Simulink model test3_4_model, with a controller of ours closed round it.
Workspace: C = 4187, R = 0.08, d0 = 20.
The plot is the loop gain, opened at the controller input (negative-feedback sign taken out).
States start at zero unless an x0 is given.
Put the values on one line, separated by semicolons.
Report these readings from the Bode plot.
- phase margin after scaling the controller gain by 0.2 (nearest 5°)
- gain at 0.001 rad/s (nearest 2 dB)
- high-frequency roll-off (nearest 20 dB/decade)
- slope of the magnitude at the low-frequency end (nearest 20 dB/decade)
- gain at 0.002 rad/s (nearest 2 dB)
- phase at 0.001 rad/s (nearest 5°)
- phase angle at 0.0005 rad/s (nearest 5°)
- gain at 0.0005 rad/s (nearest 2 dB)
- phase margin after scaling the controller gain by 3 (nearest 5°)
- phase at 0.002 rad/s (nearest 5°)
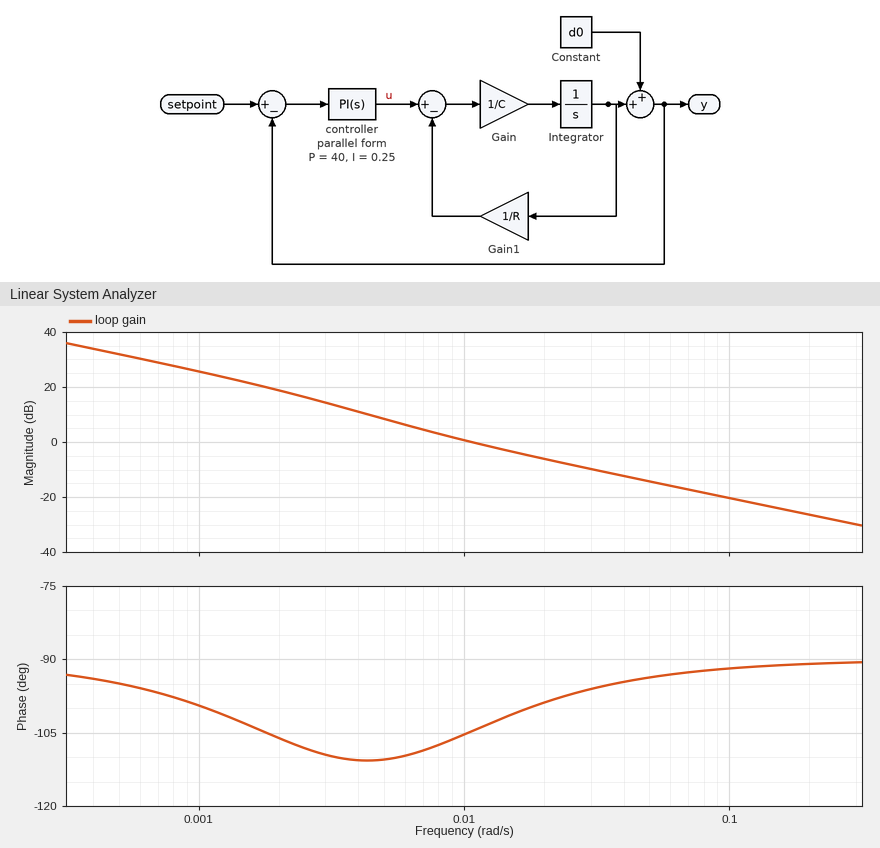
70°; 26 dB; -20 dB/decade; -20 dB/decade; 18 dB; -100°; -95°; 32 dB; 85°; -105°
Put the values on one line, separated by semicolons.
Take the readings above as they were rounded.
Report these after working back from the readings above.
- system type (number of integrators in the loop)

1
